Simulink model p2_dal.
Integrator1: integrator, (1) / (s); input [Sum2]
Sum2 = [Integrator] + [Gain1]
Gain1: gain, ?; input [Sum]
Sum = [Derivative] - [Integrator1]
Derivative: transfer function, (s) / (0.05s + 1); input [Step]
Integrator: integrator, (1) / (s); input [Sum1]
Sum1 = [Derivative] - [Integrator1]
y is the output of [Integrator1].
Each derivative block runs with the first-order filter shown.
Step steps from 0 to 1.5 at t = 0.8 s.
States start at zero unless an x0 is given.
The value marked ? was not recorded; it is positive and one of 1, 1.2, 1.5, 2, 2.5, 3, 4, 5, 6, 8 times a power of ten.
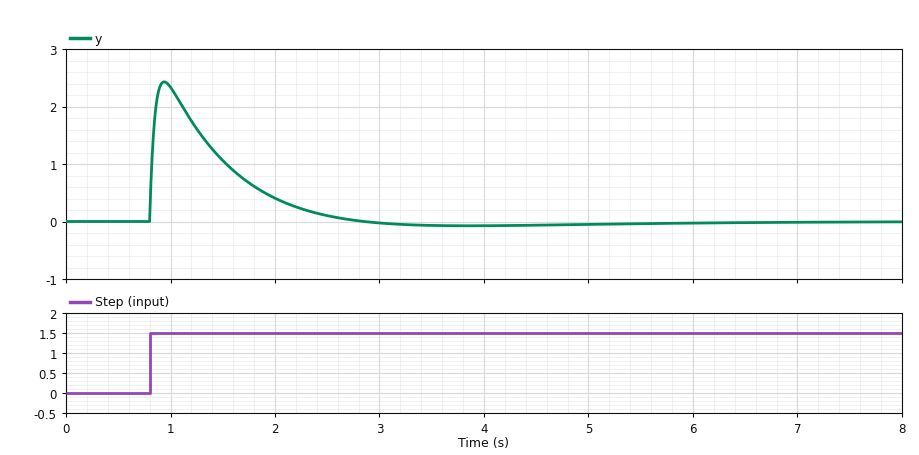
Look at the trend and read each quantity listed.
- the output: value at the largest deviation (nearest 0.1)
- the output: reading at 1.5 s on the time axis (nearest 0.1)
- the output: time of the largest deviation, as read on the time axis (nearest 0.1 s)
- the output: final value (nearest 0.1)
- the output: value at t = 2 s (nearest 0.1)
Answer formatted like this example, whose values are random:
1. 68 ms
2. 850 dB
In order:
1. 2.4
2. 1.1
3. 0.9 s
4. 0.0
5. 0.4
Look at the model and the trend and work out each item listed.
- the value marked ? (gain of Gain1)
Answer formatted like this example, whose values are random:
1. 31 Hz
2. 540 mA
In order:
1. 2
